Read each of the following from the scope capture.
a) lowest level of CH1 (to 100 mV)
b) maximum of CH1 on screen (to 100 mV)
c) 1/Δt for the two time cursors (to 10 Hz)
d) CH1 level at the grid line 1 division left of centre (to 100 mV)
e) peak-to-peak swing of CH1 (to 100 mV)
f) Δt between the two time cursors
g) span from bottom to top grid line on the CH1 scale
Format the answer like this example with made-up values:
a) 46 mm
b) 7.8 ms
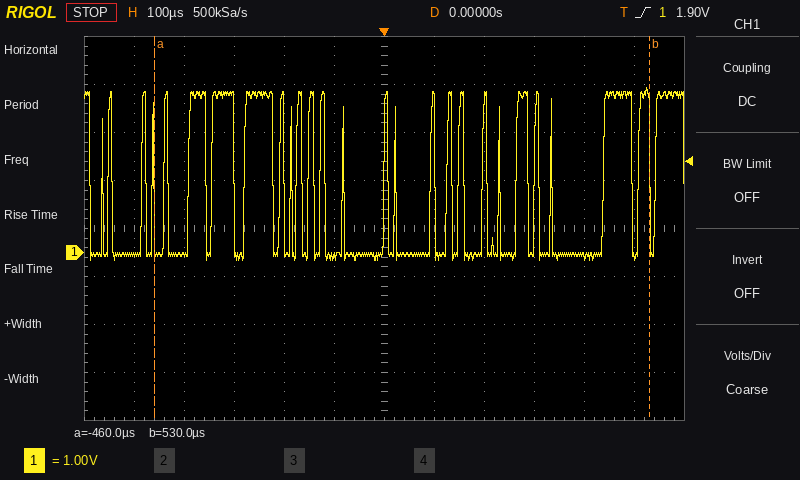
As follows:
a) -200 mV
b) 3.4 V
c) 1.01 kHz
d) -100 mV
e) 3.6 V
f) 990 µs
g) 8 V
